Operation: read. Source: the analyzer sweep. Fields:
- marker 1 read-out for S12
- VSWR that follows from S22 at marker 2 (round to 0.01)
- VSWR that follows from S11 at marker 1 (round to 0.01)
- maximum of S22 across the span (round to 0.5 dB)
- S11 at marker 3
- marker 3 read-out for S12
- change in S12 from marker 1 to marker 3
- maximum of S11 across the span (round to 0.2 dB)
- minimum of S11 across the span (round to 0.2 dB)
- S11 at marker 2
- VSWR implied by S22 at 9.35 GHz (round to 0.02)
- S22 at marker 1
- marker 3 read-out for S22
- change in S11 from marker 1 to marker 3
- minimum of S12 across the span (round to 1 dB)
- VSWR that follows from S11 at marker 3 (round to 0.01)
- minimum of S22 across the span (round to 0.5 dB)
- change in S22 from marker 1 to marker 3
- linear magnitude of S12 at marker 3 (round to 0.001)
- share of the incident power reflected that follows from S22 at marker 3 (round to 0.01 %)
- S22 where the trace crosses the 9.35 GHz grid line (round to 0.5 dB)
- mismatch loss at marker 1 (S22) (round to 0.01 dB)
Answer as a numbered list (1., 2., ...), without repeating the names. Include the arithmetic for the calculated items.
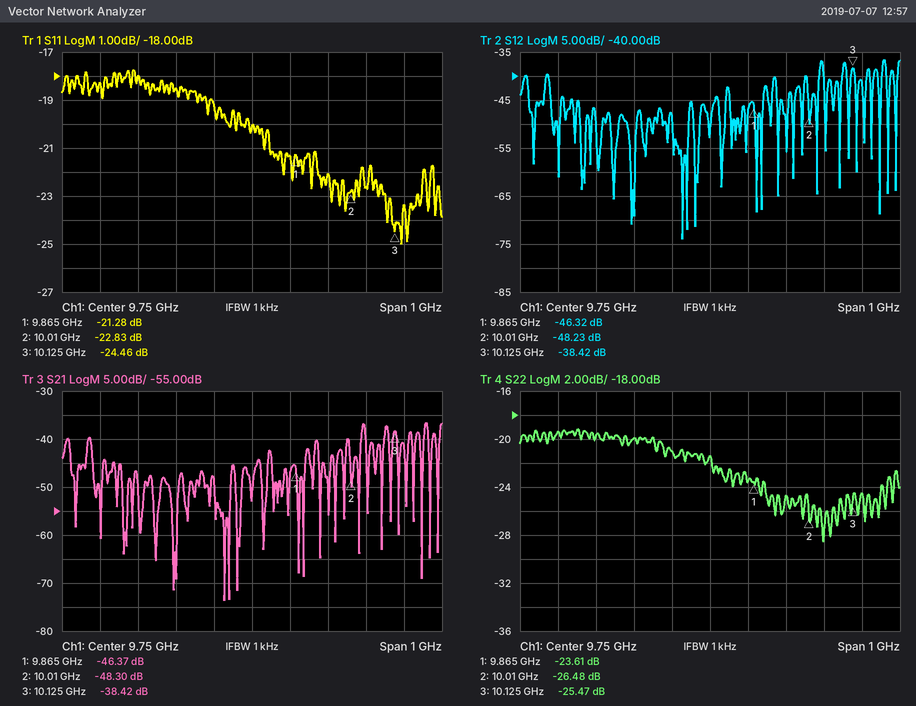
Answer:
1. -46.32 dB
2. (1 + 0.0474)/(1 − 0.0474) ≈ 1.10
3. (1 + 0.0863)/(1 − 0.0863) ≈ 1.19
4. -19.0 dB
5. -24.46 dB
6. -38.42 dB
7. -38.42 − (-46.32) = 7.90 dB
8. -17.8 dB
9. -25.0 dB
10. -22.83 dB
11. |Γ| = 10^(-19.5/20) = 0.1059; VSWR = (1 + 0.1059)/(1 − 0.1059) ≈ 1.24
12. -23.61 dB
13. -25.47 dB
14. -24.46 − (-21.28) = -3.18 dB
15. -74 dB
16. (1 + 0.0598)/(1 − 0.0598) ≈ 1.13
17. -28.5 dB
18. -25.47 − (-23.61) = -1.86 dB
19. 10^(-38.42/20) ≈ 0.012
20. 10^(-25.47/10) ≈ 0.28 %
21. -19.5 dB
22. −10 log10(1 − 10^(-23.61/10)) ≈ 0.02 dB
